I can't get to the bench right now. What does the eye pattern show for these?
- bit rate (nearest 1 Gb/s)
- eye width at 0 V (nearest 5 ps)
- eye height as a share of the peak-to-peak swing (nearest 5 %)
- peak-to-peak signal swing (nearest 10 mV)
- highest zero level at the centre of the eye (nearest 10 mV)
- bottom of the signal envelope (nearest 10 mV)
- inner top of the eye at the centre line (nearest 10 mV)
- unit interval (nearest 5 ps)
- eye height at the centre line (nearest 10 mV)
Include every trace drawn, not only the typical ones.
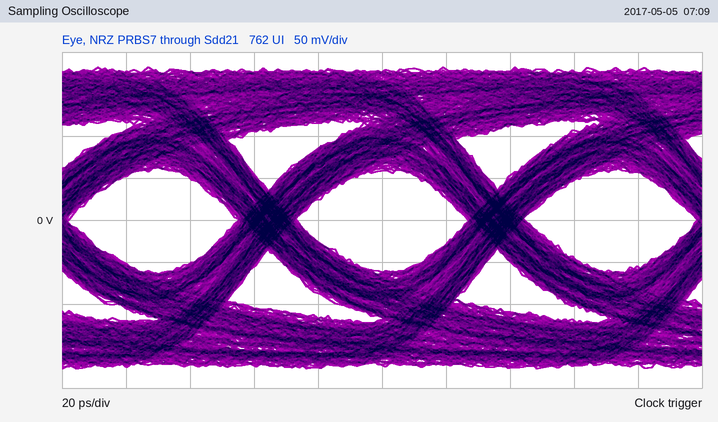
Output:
14 Gb/s
55 ps
35 %
360 mV
-60 mV
-180 mV
60 mV
70 ps
120 mV
